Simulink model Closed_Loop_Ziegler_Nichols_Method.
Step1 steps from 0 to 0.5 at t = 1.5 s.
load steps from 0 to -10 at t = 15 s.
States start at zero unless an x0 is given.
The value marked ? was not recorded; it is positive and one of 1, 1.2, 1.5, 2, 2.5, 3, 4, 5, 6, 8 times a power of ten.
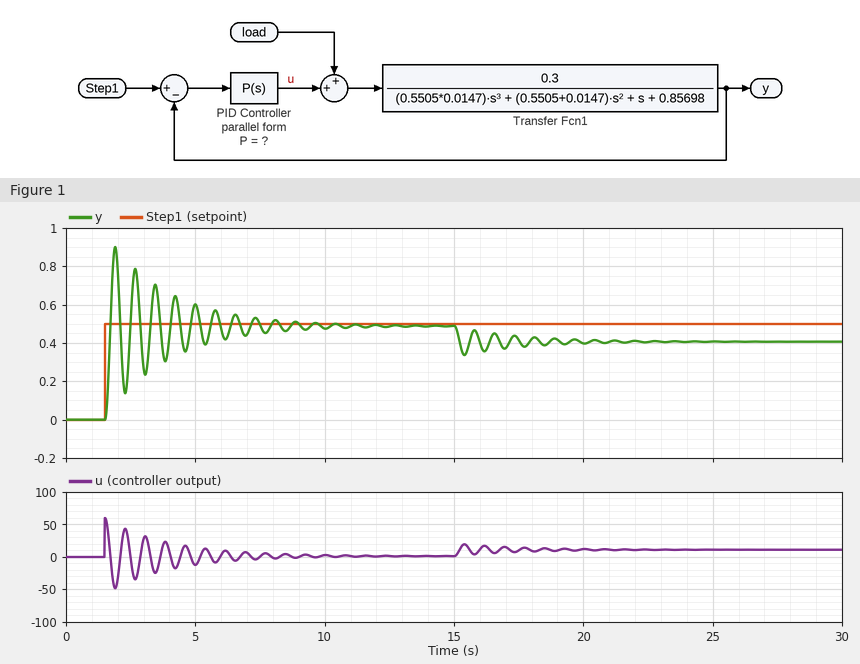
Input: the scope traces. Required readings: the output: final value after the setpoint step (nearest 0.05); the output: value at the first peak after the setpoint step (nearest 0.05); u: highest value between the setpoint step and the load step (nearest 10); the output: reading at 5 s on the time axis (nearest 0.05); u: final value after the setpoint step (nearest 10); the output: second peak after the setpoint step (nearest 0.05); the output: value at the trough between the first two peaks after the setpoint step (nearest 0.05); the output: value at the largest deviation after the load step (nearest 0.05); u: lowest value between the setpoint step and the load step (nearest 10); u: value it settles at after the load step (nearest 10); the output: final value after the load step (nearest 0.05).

0.50
0.90
60
0.60
0
0.80
0.15
0.35
-50
10
0.40
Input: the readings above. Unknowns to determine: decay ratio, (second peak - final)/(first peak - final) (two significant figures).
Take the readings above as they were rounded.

0.75
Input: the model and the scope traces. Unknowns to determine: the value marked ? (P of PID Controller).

120
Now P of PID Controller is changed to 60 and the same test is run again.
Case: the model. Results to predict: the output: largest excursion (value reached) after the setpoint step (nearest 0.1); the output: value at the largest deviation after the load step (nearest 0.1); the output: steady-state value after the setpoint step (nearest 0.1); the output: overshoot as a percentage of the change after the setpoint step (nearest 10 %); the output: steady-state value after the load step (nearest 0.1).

0.8
0.2
0.5
70 %
0.3
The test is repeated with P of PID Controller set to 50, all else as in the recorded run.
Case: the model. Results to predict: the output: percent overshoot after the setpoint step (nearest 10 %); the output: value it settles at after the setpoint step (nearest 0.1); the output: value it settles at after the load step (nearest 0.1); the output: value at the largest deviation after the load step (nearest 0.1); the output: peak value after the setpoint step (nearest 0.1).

70 %
0.5
0.3
0.2
0.8
